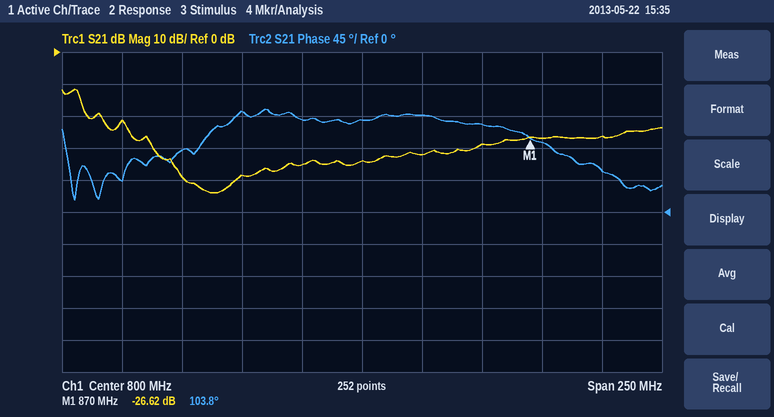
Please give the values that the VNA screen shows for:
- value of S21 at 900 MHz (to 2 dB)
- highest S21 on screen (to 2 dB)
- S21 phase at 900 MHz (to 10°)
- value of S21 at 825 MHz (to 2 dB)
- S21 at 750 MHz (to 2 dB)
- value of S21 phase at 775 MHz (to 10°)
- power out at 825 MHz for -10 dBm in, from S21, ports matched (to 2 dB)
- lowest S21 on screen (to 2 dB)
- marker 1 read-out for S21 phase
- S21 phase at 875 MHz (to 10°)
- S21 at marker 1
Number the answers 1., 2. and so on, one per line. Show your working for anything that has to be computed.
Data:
1. -26 dB
2. -12 dB
3. 60°
4. -32 dB
5. -38 dB
6. 130°
7. -10 dBm + (-32 dB) = -42 dBm
8. -44 dB
9. 103.8°
10. 100°
11. -26.62 dB
